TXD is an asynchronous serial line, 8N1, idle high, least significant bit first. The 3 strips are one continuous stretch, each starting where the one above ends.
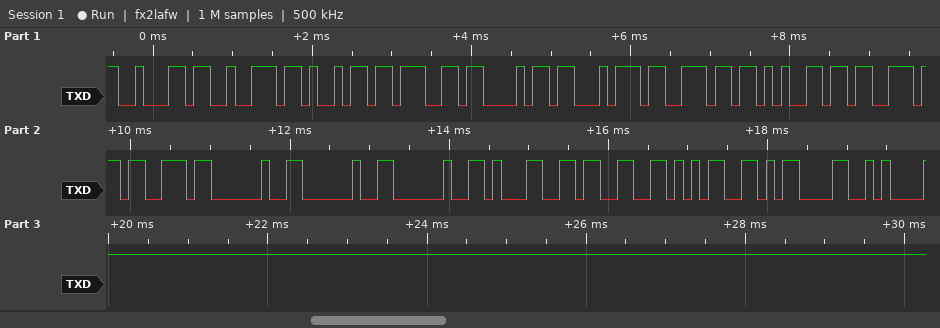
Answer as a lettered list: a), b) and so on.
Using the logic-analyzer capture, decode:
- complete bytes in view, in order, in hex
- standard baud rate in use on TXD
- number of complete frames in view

a) 0x62 0x72 0x69 0x67 0x68 0x74 0x6E 0x65 0x73 0x73 0x20 0x20 0x20 0x31 0x33 0x35 0x0D 0x0A
b) 9600 baud
c) 18
